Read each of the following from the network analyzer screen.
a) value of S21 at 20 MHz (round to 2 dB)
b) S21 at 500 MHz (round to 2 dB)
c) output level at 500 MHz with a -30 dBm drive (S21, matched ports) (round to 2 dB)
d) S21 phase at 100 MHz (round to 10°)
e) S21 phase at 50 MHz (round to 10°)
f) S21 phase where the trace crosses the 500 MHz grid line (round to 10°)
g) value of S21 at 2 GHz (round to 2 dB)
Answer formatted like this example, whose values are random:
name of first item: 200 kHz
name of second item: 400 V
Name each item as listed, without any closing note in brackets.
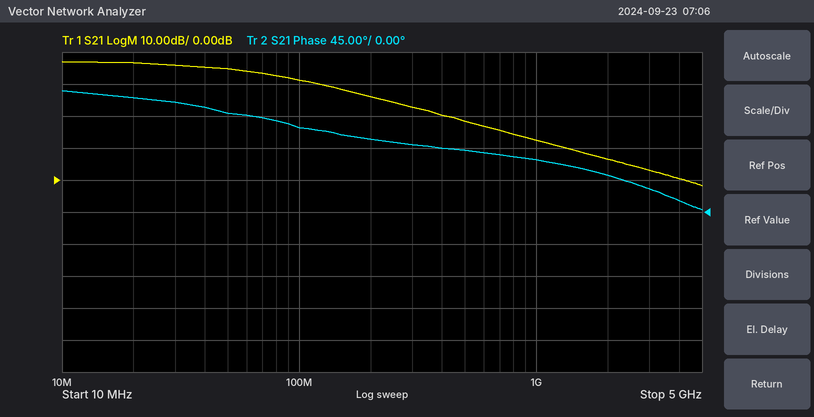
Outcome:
value of S21 at 20 MHz: 36 dB
S21 at 500 MHz: 18 dB
output level at 500 MHz with a -30 dBm drive (S21, matched ports): -12 dBm
S21 phase at 100 MHz: 120°
S21 phase at 50 MHz: 140°
S21 phase where the trace crosses the 500 MHz grid line: 90°
value of S21 at 2 GHz: 6 dB
